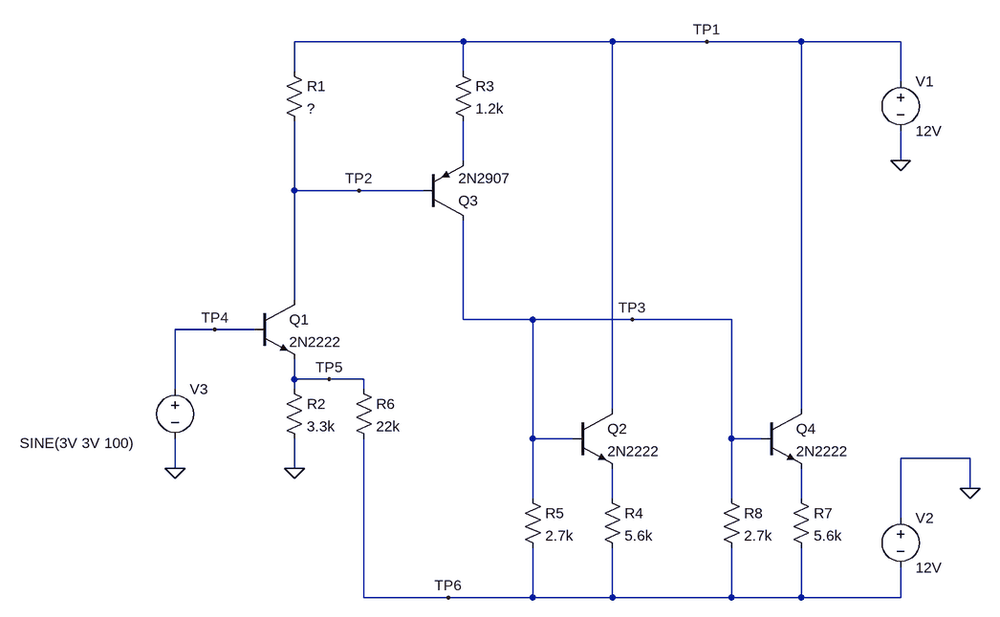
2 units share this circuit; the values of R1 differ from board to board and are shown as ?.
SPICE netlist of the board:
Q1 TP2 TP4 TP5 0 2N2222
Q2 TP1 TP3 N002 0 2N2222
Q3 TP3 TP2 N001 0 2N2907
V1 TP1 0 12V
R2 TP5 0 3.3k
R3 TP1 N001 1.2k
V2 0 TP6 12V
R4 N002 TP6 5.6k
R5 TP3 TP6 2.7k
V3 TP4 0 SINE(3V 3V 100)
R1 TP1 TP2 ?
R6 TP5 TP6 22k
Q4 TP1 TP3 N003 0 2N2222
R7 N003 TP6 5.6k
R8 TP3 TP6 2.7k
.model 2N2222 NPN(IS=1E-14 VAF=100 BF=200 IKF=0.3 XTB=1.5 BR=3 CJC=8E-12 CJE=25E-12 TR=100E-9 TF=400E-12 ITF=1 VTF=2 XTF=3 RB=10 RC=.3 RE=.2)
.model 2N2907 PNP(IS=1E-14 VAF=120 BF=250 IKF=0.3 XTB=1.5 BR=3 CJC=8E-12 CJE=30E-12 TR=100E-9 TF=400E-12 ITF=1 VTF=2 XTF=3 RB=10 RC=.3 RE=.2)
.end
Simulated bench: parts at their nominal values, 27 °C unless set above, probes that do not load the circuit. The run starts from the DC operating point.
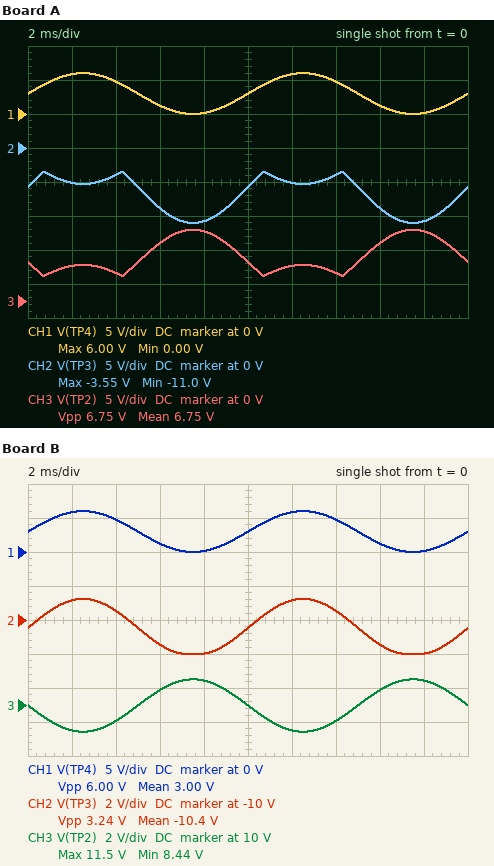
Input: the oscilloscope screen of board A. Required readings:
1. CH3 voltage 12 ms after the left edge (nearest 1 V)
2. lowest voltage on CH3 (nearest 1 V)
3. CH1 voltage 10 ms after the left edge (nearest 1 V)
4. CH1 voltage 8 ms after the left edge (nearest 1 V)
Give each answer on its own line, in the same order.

5 V
4 V
3 V
0 V
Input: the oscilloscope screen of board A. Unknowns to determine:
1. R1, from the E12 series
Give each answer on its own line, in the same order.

4.7 kΩ
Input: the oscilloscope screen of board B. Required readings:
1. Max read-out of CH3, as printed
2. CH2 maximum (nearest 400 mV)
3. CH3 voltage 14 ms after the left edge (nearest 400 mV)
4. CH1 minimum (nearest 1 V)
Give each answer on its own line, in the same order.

11.5 V
-8.8 V
9.2 V
0 V
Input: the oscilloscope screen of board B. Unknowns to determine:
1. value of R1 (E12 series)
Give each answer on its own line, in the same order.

1.5 kΩ
